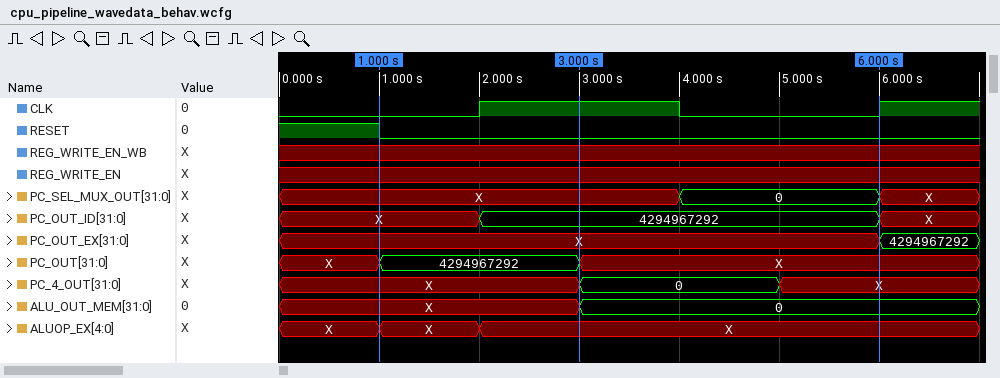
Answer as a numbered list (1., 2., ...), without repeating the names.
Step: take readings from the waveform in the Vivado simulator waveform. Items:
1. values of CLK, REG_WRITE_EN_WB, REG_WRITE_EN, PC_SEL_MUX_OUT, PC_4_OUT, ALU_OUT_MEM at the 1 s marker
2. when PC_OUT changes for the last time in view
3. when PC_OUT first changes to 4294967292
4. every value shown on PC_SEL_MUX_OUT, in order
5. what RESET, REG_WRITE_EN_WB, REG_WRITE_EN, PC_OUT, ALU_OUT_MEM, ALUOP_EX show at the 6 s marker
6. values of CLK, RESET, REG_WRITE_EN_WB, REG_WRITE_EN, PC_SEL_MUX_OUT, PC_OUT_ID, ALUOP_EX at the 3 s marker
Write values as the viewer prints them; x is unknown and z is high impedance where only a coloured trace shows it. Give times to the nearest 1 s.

1. CLK=0, REG_WRITE_EN_WB=x, REG_WRITE_EN=x, PC_SEL_MUX_OUT=X, PC_4_OUT=X, ALU_OUT_MEM=X
2. 3 s
3. 1 s
4. X, 0, X
5. RESET=0, REG_WRITE_EN_WB=x, REG_WRITE_EN=x, PC_OUT=X, ALU_OUT_MEM=0, ALUOP_EX=X
6. CLK=1, RESET=0, REG_WRITE_EN_WB=x, REG_WRITE_EN=x, PC_SEL_MUX_OUT=X, PC_OUT_ID=4294967292, ALUOP_EX=X
